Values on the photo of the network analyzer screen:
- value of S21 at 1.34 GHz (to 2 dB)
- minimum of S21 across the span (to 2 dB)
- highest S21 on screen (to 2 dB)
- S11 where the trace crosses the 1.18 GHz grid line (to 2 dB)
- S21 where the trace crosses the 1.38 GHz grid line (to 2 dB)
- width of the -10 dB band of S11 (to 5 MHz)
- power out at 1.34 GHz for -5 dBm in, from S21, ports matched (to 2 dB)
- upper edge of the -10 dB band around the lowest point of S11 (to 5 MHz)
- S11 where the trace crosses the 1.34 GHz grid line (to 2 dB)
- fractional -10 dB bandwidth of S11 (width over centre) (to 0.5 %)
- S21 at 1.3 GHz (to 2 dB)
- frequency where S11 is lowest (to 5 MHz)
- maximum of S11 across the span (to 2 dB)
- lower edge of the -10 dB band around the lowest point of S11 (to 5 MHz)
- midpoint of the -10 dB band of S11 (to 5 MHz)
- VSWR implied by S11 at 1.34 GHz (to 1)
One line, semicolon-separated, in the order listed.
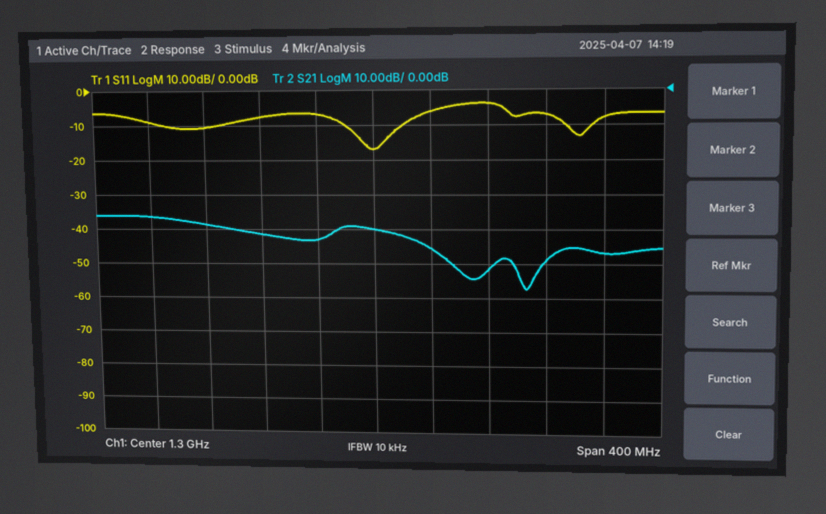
-46 dB; -58 dB; -36 dB; -10 dB; -52 dB; 40 MHz; -50 dBm; 1.320 GHz; -6 dB; 3.0 %; -40 dB; 1.300 GHz; -4 dB; 1.280 GHz; 1.300 GHz; 3
